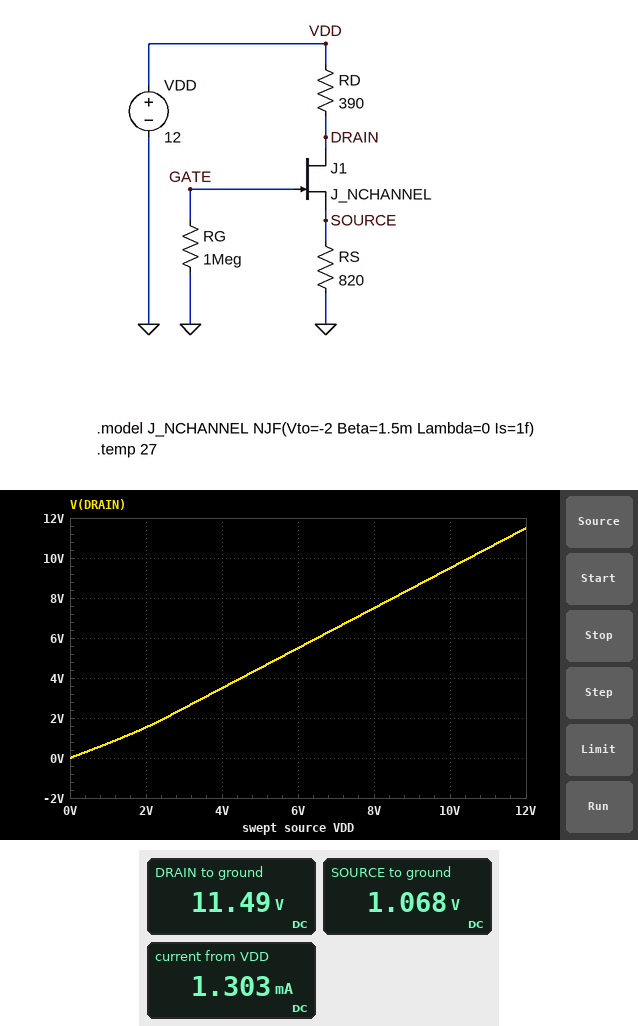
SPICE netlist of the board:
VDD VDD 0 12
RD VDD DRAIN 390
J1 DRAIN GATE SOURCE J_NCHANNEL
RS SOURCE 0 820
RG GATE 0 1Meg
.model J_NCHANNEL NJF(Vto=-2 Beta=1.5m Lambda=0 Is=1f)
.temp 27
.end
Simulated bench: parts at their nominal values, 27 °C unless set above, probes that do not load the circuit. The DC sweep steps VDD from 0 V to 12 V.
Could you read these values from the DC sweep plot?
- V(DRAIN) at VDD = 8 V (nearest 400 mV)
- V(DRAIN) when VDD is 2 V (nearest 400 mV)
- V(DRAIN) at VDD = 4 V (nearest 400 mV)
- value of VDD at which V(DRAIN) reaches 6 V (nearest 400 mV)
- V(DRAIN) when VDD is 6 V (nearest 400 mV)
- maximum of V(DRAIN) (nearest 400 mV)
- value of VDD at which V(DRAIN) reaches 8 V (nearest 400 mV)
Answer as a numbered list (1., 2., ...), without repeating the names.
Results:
1. 7.6 V
2. 1.6 V
3. 3.6 V
4. 6.4 V
5. 5.6 V
6. 11.6 V
7. 8.4 V
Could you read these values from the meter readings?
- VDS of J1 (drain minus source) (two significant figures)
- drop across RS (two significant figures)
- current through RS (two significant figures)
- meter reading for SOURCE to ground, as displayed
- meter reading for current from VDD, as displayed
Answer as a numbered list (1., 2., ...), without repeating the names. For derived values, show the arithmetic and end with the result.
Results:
1. 11.49 V - 1.068 V = 10 V
2. 1.068 V = 1.1 V
3. (1.068 V) / 820 Ω = 1.3 mA
4. 1.068 V
5. 1.303 mA
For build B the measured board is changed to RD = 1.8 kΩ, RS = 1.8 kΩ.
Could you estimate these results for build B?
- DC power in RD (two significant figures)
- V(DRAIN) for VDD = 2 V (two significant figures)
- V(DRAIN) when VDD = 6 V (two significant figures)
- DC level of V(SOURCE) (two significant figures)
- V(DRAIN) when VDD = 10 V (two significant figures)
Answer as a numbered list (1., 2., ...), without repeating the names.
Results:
1. 950 µW
2. 1.1 V
3. 4.7 V
4. 1.3 V
5. 8.7 V
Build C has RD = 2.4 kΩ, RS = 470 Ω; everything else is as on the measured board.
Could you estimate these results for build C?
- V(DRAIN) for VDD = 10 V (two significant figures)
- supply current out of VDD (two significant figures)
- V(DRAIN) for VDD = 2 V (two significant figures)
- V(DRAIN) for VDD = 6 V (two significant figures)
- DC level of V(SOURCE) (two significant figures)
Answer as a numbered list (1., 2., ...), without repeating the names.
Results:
1. 5.5 V
2. 1.9 mA
3. 440 mV
4. 1.7 V
5. 880 mV
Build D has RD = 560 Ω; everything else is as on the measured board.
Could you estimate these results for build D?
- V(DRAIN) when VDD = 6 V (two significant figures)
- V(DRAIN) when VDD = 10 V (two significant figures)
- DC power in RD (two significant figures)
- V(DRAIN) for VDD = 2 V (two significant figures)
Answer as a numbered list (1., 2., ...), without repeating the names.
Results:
1. 5.3 V
2. 9.3 V
3. 950 µW
4. 1.4 V
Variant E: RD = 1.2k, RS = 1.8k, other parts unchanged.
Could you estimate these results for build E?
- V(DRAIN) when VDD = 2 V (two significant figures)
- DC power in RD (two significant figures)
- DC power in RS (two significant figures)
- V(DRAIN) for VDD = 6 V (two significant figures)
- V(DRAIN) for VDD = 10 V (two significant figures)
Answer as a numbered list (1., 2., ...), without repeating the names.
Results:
1. 1.3 V
2. 630 µW
3. 950 µW
4. 5.1 V
5. 9.1 V
